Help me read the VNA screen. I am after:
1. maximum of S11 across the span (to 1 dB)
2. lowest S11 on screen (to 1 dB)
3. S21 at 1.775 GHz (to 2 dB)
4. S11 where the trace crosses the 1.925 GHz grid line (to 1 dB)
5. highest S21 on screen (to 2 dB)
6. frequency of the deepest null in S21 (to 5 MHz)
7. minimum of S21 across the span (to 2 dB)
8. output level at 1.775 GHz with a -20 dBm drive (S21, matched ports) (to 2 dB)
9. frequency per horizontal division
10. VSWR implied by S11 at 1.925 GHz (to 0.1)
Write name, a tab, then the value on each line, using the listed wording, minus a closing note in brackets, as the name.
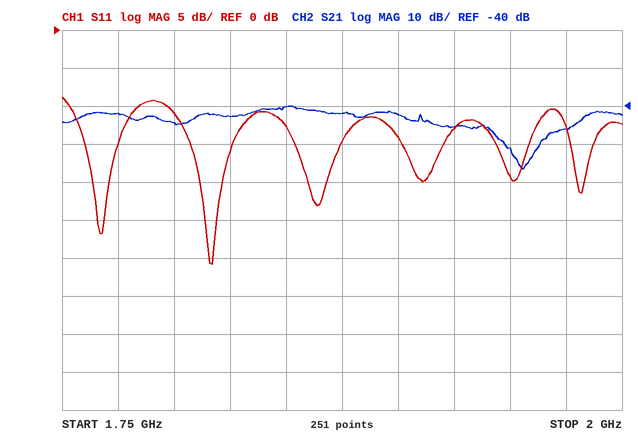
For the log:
maximum of S11 across the span	-9 dB
lowest S11 on screen	-31 dB
S21 at 1.775 GHz	-42 dB
S11 where the trace crosses the 1.925 GHz grid line	-13 dB
highest S21 on screen	-40 dB
frequency of the deepest null in S21	1.955 GHz
minimum of S21 across the span	-56 dB
output level at 1.775 GHz with a -20 dBm drive (S21, matched ports)	-62 dBm
frequency per horizontal division	25 MHz
VSWR implied by S11 at 1.925 GHz	1.6
